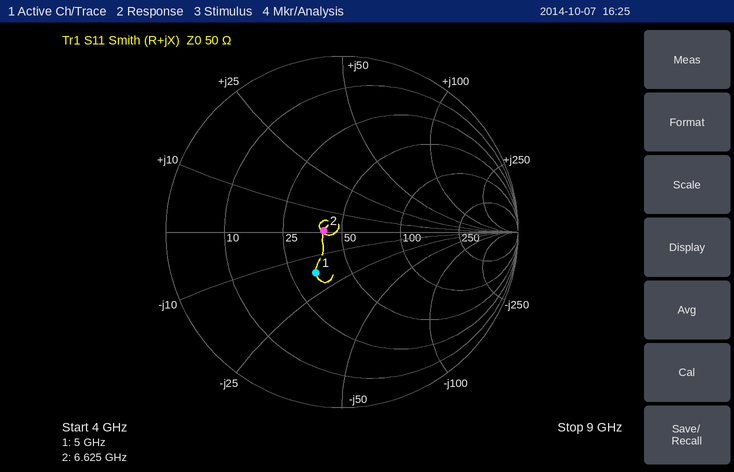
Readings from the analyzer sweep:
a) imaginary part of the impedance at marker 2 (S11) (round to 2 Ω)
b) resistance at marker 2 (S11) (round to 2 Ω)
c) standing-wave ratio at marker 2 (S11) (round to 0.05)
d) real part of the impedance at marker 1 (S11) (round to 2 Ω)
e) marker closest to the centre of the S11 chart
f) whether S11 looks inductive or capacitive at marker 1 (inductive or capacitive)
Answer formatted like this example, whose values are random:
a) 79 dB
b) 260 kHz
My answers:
a) 0 Ω
b) 40 Ω
c) 1.25
d) 34 Ω
e) marker 2
f) capacitive
